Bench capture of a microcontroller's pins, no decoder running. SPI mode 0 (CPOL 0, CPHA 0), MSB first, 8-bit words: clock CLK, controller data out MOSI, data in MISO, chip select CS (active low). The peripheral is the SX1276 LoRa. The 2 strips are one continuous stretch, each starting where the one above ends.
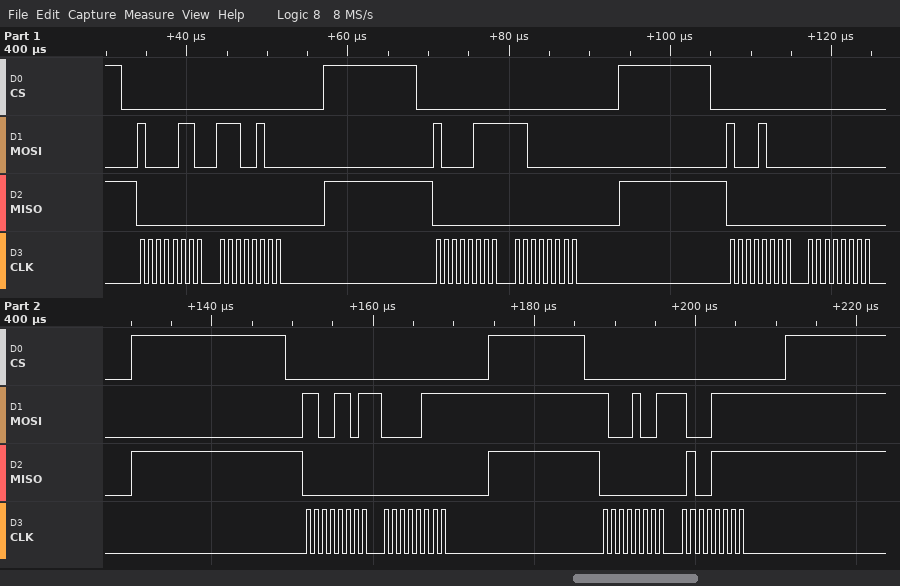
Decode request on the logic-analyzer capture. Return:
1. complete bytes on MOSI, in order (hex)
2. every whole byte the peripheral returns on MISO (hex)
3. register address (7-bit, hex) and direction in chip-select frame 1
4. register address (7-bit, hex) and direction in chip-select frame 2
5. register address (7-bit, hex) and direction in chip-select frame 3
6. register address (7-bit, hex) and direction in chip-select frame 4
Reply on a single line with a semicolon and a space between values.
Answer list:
86 E4 87 C0 88 00 CD 07 89 8F; 00 00 00 00 00 00 00 00 00 4F; 0x06 write; 0x07 write; 0x08 write; 0x4D write
